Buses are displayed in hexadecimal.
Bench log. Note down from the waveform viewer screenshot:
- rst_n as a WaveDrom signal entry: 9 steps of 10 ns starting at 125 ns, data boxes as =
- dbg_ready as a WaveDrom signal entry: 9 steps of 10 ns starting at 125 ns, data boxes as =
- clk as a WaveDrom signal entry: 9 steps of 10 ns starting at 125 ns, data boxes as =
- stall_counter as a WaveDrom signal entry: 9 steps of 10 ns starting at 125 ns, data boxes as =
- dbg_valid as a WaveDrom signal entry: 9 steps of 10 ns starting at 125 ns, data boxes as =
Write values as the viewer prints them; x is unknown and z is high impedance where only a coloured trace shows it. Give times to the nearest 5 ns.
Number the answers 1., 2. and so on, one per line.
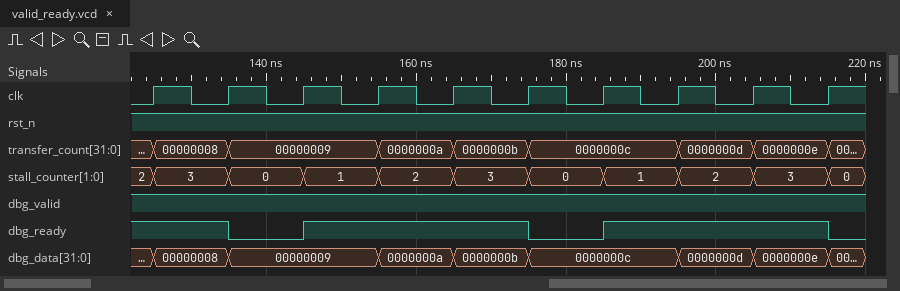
1. {name: 'rst_n', wave: '1........'}
2. {name: 'dbg_ready', wave: '101..01..'}
3. {name: 'clk', wave: 'p........'}
4. {name: 'stall_counter', wave: '=========', data: '3 0 1 2 3 0 1 2 3'}
5. {name: 'dbg_valid', wave: '1........'}
